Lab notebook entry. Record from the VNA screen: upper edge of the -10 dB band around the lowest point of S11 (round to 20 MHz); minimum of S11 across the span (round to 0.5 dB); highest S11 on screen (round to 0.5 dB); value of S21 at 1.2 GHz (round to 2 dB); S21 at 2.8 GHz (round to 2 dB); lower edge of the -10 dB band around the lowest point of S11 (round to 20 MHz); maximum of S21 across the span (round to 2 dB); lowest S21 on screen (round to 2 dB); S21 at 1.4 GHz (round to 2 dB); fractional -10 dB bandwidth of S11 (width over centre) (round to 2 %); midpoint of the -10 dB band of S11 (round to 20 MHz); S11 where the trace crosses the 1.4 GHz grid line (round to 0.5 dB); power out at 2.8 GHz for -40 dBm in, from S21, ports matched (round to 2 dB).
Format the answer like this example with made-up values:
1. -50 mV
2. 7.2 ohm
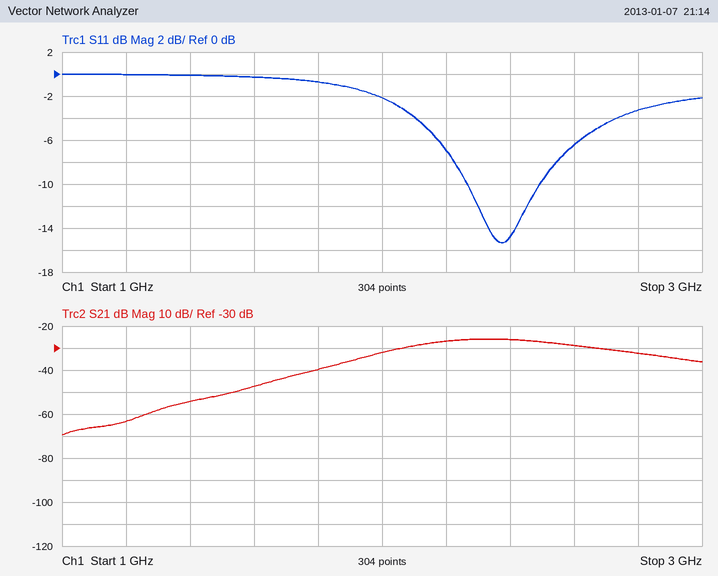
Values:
1. 2.50 GHz
2. -15.5 dB
3. 0.0 dB
4. -64 dB
5. -32 dB
6. 2.26 GHz
7. -26 dB
8. -70 dB
9. -54 dB
10. 10 %
11. 2.38 GHz
12. 0.0 dB
13. -72 dBm
